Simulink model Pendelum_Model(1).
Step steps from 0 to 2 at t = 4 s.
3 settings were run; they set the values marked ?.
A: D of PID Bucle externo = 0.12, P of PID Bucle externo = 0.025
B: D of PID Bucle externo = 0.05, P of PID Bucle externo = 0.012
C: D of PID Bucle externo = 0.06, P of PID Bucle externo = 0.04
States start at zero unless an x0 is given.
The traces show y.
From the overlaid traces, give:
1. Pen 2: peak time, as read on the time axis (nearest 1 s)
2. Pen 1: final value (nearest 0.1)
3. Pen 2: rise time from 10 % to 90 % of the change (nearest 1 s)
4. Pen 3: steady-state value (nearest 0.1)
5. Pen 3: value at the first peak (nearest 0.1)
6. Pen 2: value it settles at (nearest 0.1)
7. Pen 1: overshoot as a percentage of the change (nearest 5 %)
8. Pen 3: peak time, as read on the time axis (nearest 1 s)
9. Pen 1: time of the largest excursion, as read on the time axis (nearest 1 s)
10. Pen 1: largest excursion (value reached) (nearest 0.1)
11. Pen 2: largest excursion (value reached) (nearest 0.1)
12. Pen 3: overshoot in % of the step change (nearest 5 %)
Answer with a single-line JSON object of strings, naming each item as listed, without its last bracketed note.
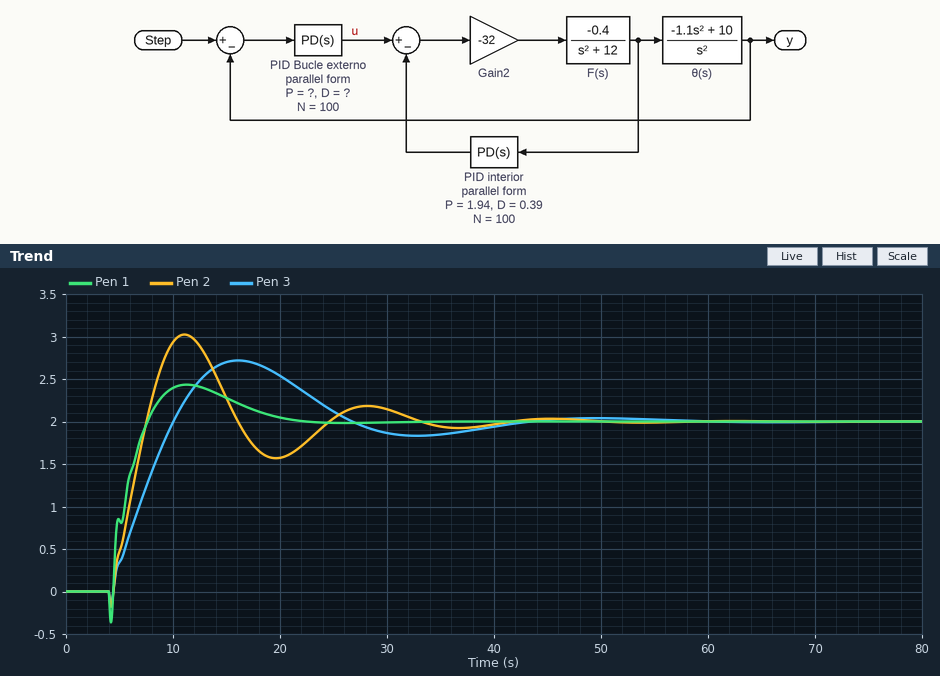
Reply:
{"Pen 2: peak time, as read on the time axis": "11 s", "Pen 1: final value": "2.0", "Pen 2: rise time from 10 % to 90 % of the change": "3 s", "Pen 3: steady-state value": "2.0", "Pen 3: value at the first peak": "2.7", "Pen 2: value it settles at": "2.0", "Pen 1: overshoot as a percentage of the change": "20 %", "Pen 3: peak time, as read on the time axis": "16 s", "Pen 1: time of the largest excursion, as read on the time axis": "11 s", "Pen 1: largest excursion (value reached)": "2.4", "Pen 2: largest excursion (value reached)": "3.0", "Pen 3: overshoot in % of the step change": "35 %"}
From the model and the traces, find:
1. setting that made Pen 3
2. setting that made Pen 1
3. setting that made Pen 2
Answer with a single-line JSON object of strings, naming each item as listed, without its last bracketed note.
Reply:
{"setting that made Pen 3": "B", "setting that made Pen 1": "A", "setting that made Pen 2": "C"}
